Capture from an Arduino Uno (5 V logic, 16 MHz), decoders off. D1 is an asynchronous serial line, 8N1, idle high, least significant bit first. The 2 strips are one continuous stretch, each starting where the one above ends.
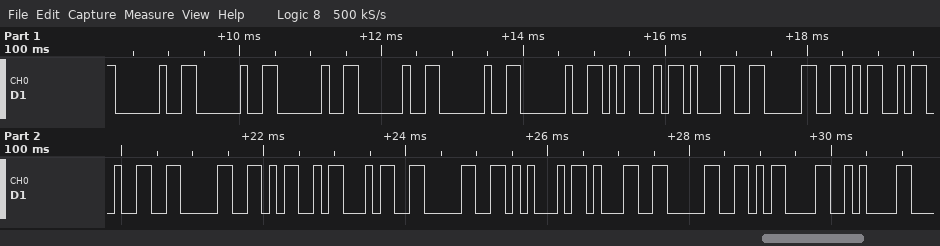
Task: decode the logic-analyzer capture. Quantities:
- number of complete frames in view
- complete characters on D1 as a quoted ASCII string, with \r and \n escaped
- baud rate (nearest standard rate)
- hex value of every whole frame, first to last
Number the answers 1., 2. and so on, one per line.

1. 20
2. "      M10M20M40E10\r\n"
3. 9600 baud
4. 20 20 20 20 20 20 4D 31 30 4D 32 30 4D 34 30 45 31 30 0D 0A
